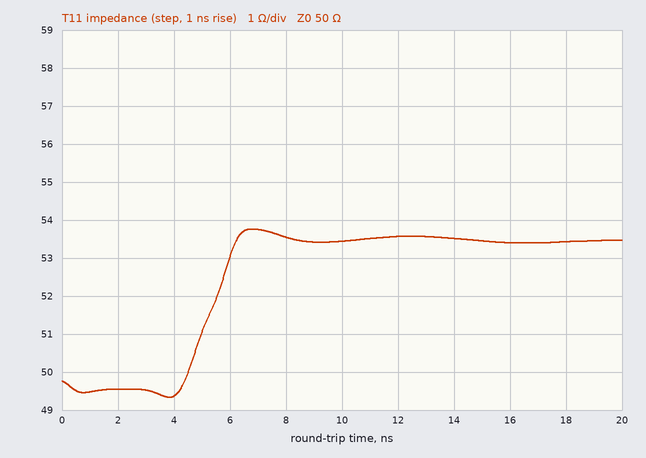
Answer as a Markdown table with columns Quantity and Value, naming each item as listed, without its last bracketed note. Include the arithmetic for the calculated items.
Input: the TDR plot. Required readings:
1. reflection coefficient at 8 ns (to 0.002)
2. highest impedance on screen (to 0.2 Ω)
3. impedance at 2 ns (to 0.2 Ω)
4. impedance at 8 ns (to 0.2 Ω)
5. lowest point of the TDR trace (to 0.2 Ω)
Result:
| Quantity | Value |
|---|---|
| reflection coefficient at 8 ns | (53.6 − 50)/(53.6 + 50) ≈ +0.0347, so +0.034 to the nearest 0.002 |
| highest impedance on screen | 53.8 Ω |
| impedance at 2 ns | 49.6 Ω |
| impedance at 8 ns | 53.6 Ω |
| lowest point of the TDR trace | 49.4 Ω |
